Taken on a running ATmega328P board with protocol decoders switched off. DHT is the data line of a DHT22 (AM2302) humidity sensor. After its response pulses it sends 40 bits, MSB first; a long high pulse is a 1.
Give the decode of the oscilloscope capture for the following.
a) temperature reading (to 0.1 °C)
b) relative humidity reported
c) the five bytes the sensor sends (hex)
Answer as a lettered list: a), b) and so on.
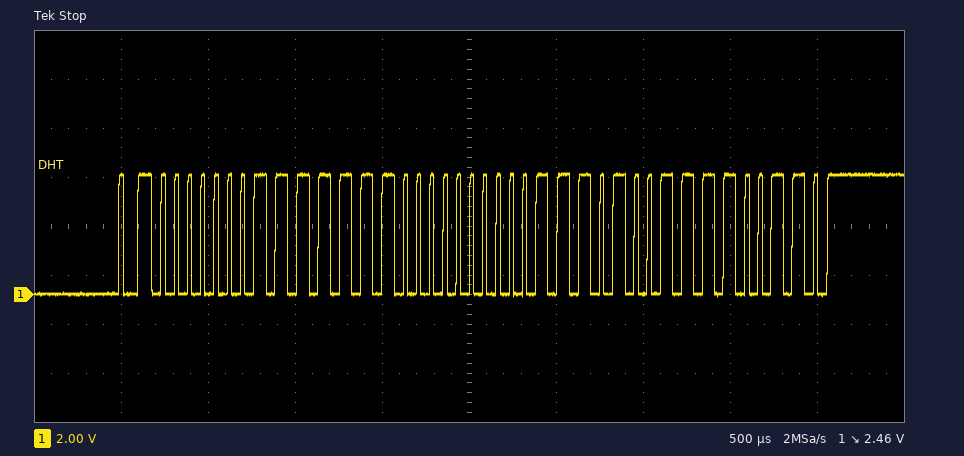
a) 23.3 °C
b) 50.8 %
c) 01 FC 00 E9 E6
